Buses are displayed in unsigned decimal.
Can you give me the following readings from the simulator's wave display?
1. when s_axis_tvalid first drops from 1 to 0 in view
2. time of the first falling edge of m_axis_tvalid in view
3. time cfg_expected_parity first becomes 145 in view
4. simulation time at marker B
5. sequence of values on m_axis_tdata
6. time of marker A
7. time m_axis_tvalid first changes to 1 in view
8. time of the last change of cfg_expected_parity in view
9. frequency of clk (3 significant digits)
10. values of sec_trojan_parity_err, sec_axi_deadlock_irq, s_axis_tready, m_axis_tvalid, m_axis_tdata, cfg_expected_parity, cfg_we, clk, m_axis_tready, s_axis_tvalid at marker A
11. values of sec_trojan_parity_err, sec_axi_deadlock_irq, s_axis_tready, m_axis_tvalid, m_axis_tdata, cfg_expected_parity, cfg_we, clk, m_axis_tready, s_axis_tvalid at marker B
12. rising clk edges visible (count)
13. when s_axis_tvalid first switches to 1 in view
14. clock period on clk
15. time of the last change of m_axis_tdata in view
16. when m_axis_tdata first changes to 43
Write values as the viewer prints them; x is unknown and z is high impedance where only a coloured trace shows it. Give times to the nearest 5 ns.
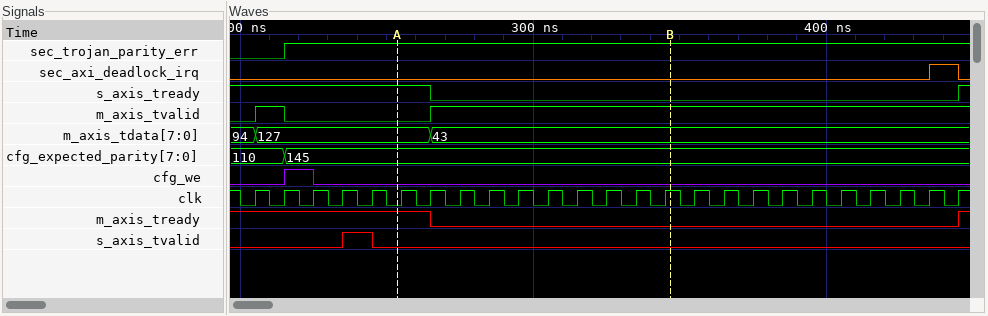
245 ns
215 ns
215 ns
345 ns
94, 127, 43
255 ns
205 ns
215 ns
100 MHz
sec_trojan_parity_err=1, sec_axi_deadlock_irq=0, s_axis_tready=1, m_axis_tvalid=0, m_axis_tdata=127, cfg_expected_parity=145, cfg_we=0, clk=0, m_axis_tready=1, s_axis_tvalid=0
sec_trojan_parity_err=1, sec_axi_deadlock_irq=0, s_axis_tready=0, m_axis_tvalid=1, m_axis_tdata=43, cfg_expected_parity=145, cfg_we=0, clk=1, m_axis_tready=0, s_axis_tvalid=0
25
235 ns
10 ns
265 ns
265 ns
